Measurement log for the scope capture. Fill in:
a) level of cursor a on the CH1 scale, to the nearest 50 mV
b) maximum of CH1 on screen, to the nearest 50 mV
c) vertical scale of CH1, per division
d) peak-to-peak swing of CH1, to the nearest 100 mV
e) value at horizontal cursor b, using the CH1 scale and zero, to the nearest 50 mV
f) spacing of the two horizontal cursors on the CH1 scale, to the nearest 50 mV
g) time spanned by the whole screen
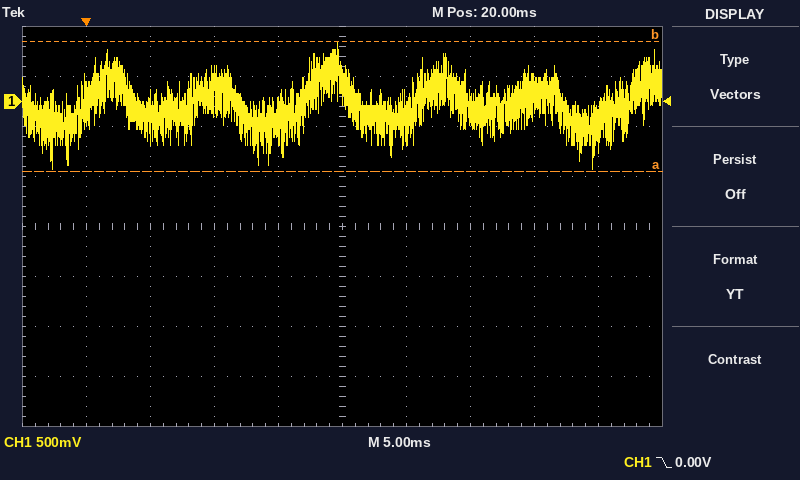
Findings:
-700 mV
600 mV
500 mV
1.30 V
600 mV
1.30 V
50 ms
